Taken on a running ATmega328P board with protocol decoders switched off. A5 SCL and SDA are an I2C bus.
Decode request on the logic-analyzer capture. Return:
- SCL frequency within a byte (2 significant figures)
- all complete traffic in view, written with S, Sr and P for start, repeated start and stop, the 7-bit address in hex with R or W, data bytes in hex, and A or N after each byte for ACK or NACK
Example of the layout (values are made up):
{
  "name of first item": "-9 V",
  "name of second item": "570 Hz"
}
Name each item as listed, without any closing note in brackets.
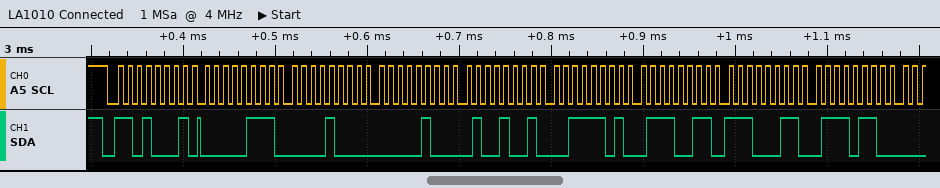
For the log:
{
  "SCL frequency within a byte": "100 kHz",
  "all complete traffic in view, written with S, Sr and P for start, repeated start and stop, the 7-bit address in hex with R or W, data bytes in hex, and A or N after each byte for ACK or NACK": "S 68R A 07 A 08 A 04 A 49 A 3D A 73 A E3 A 76 A"
}
